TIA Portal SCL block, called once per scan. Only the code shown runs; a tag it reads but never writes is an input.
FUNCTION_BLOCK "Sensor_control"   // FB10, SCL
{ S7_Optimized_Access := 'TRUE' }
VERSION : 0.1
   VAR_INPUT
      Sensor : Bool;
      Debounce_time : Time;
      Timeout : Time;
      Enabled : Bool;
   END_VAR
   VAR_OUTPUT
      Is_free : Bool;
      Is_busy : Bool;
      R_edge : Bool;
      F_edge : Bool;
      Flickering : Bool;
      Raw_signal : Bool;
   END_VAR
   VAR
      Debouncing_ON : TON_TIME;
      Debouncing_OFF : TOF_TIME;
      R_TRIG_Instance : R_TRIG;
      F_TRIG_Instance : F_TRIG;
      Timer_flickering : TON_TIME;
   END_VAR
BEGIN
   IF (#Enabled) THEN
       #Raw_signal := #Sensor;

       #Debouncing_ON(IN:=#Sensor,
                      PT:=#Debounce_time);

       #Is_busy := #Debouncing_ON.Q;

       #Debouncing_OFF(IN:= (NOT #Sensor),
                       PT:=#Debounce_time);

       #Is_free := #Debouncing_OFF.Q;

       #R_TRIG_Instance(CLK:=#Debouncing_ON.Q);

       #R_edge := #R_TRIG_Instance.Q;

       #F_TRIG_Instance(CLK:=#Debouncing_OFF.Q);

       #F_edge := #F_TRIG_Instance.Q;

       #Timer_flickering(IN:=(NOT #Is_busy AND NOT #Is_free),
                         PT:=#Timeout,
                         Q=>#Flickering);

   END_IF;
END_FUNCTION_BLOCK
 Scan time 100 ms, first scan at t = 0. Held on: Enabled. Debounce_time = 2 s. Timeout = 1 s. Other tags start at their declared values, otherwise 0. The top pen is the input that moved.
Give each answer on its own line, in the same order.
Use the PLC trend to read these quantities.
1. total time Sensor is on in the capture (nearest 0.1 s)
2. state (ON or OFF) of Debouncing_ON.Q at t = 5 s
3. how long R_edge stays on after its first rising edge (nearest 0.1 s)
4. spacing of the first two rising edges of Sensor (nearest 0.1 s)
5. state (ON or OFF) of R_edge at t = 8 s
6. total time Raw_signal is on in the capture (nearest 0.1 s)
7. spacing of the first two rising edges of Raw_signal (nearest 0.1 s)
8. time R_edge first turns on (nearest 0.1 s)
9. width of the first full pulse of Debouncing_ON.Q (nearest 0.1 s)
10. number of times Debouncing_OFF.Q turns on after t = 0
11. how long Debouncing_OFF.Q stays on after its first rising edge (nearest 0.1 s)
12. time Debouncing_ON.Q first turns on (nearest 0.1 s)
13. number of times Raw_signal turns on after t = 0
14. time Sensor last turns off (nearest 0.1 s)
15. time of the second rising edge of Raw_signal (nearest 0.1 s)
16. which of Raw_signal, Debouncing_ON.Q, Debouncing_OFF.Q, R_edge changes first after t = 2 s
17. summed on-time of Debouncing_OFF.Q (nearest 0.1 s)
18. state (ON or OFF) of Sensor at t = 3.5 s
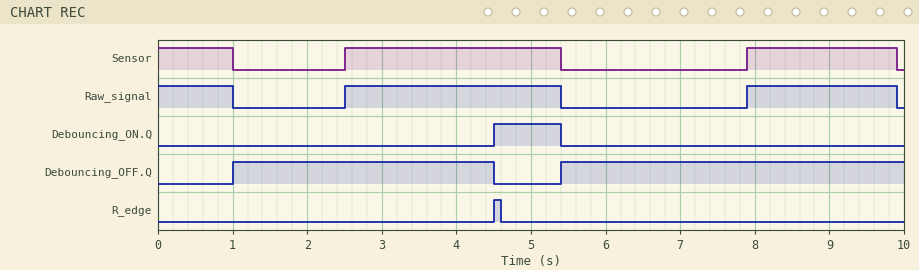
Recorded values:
5.9 s
ON
0.1 s
5.4 s
OFF
5.9 s
5.4 s
4.5 s
0.9 s
2
3.5 s
4.5 s
2
9.9 s
7.9 s
Raw_signal
8.1 s
ON
